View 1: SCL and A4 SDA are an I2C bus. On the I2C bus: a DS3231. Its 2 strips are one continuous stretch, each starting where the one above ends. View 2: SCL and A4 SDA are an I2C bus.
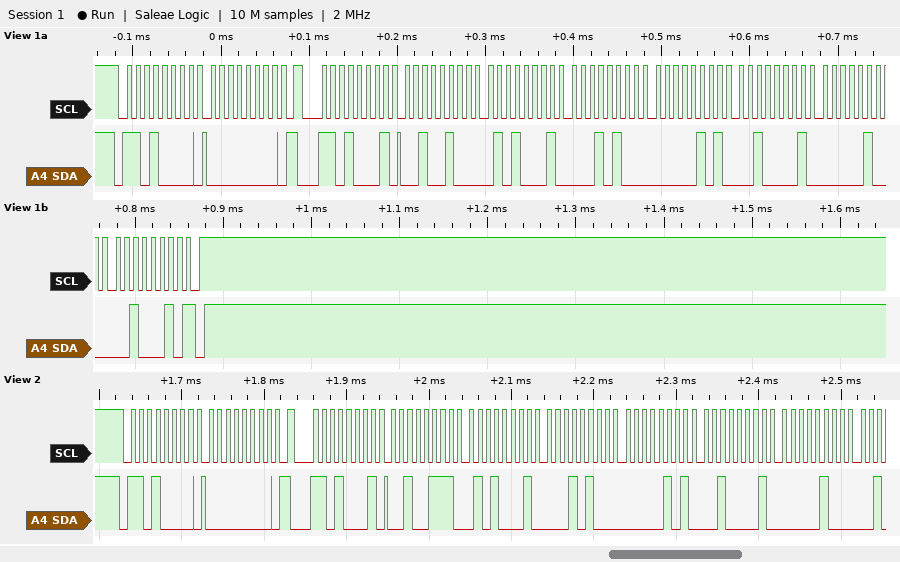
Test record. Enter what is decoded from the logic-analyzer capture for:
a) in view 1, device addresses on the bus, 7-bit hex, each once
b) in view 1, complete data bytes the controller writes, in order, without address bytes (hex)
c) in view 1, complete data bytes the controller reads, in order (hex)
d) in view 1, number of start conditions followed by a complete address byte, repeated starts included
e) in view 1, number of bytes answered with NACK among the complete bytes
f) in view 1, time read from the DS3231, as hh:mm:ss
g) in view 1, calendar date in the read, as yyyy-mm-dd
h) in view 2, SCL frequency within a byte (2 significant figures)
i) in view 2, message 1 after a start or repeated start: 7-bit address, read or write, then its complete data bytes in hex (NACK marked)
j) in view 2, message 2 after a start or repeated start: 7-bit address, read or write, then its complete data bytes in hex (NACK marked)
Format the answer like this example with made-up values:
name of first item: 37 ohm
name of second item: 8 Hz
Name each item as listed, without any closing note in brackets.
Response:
in view 1, device addresses on the bus, 7-bit hex, each once: 0x68
in view 1, complete data bytes the controller writes, in order, without address bytes: 00
in view 1, complete data bytes the controller reads, in order: 24 51 14 05 21 04 22
in view 1, number of start conditions followed by a complete address byte, repeated starts included: 2
in view 1, number of bytes answered with NACK among the complete bytes: 1
in view 1, time read from the DS3231, as hh:mm:ss: 14:51:24
in view 1, calendar date in the read, as yyyy-mm-dd: 2022-04-21
in view 2, SCL frequency within a byte: 100 kHz
in view 2, message 1 after a start or repeated start: 7-bit address, read or write, then its complete data bytes in hex: 0x68 write: 00
in view 2, message 2 after a start or repeated start: 7-bit address, read or write, then its complete data bytes in hex: 0x68 read: 27 51 14 05 21 04
